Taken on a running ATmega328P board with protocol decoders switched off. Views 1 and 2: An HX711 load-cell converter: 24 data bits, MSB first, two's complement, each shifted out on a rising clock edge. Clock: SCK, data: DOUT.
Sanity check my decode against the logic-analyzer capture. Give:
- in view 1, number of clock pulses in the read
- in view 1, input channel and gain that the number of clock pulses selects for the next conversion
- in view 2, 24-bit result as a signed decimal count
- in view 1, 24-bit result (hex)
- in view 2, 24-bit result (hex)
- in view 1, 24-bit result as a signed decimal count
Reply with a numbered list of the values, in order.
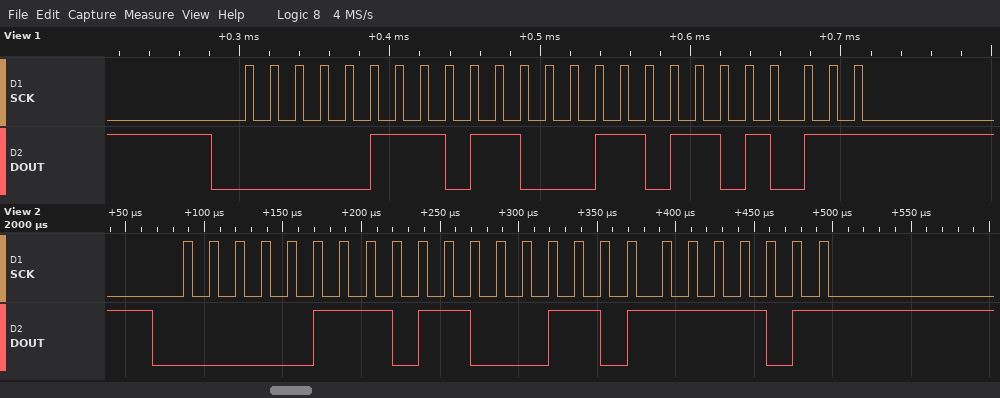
1. 25
2. channel A, gain 128
3. 484221
4. 0x07636B
5. 0x07637D
6. 484203
